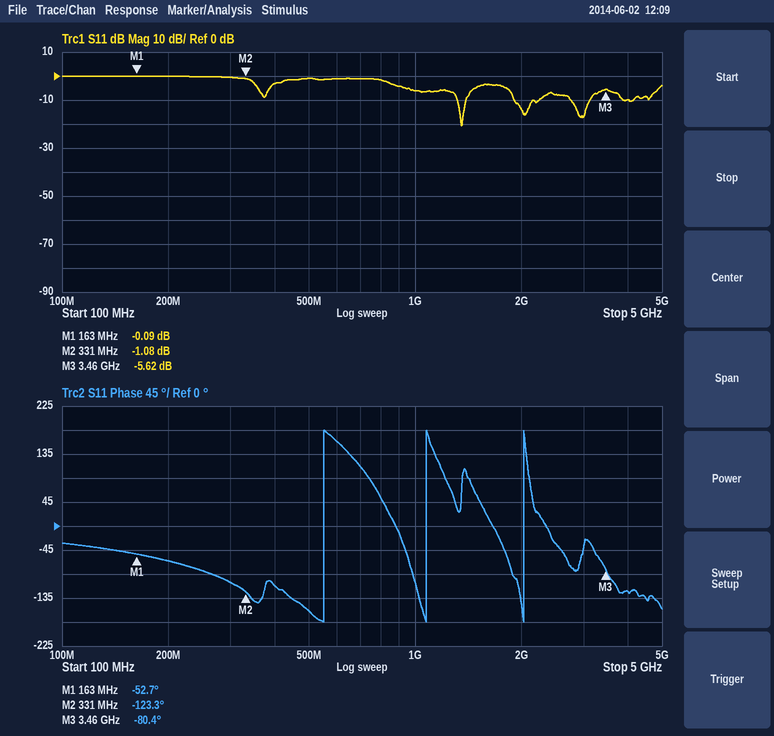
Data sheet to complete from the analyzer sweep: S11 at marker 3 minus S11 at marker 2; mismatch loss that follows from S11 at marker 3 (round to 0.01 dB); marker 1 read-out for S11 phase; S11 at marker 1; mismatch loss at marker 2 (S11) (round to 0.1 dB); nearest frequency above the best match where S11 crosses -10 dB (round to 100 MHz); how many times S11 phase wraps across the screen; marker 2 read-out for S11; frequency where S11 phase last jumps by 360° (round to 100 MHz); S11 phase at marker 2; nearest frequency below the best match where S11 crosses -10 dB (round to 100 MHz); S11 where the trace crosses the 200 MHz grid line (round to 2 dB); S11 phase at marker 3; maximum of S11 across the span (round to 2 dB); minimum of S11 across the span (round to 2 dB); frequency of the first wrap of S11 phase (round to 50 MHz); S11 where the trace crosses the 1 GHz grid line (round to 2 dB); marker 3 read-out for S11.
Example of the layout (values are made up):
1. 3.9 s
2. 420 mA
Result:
1. -4.54 dB
2. 1.39 dB
3. -52.7°
4. -0.09 dB
5. 6.6 dB
6. 1.4 GHz
7. 3
8. -1.08 dB
9. 2.0 GHz
10. -123.3°
11. 1.3 GHz
12. 0 dB
13. -80.4°
14. 0 dB
15. -20 dB
16. 550 MHz
17. -6 dB
18. -5.62 dB
